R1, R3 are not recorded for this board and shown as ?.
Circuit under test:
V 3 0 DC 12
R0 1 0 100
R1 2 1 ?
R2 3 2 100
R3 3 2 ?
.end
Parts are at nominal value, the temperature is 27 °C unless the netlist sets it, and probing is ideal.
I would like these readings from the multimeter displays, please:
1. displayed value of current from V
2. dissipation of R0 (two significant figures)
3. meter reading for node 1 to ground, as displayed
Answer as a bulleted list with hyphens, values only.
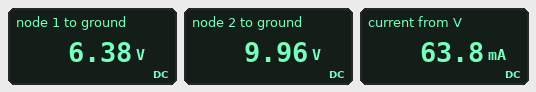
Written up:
- 63.8 mA
- 410 mW
- 6.38 V
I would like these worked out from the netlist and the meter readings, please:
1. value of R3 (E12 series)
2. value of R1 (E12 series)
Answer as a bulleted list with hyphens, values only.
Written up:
- 47 Ω
- 56 Ω
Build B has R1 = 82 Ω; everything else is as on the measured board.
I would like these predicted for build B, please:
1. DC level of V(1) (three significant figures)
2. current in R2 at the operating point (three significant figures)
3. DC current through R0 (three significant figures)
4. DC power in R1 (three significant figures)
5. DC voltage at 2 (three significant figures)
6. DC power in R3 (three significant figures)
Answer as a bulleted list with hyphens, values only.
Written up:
- 5.61 V
- 17.9 mA
- 56.1 mA
- 258 mW
- 10.2 V
- 68.4 mW
